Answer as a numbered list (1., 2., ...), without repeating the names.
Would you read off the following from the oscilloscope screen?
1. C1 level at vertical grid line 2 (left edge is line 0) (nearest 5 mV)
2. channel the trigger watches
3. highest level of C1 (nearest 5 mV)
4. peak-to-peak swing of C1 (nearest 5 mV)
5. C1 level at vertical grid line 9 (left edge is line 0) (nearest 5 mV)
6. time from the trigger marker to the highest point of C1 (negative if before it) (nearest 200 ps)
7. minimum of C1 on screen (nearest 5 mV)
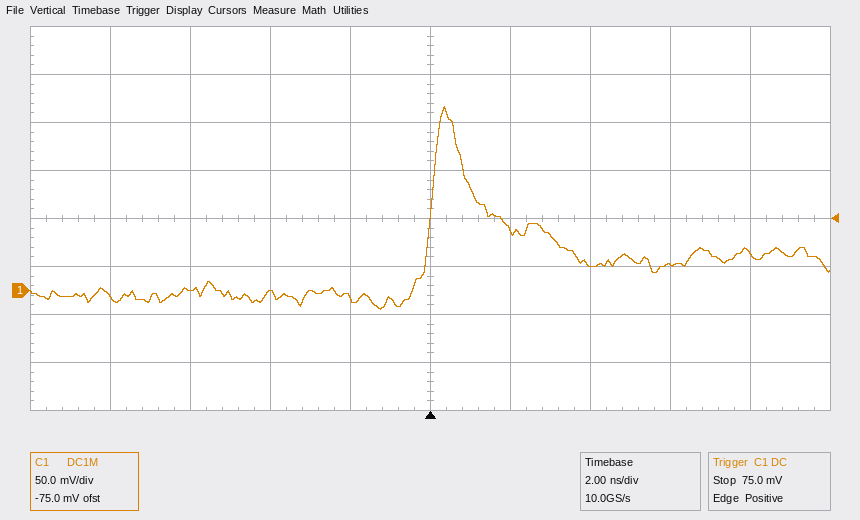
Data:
1. 0 mV
2. C1
3. 190 mV
4. 210 mV
5. 40 mV
6. +400 ps
7. -20 mV
